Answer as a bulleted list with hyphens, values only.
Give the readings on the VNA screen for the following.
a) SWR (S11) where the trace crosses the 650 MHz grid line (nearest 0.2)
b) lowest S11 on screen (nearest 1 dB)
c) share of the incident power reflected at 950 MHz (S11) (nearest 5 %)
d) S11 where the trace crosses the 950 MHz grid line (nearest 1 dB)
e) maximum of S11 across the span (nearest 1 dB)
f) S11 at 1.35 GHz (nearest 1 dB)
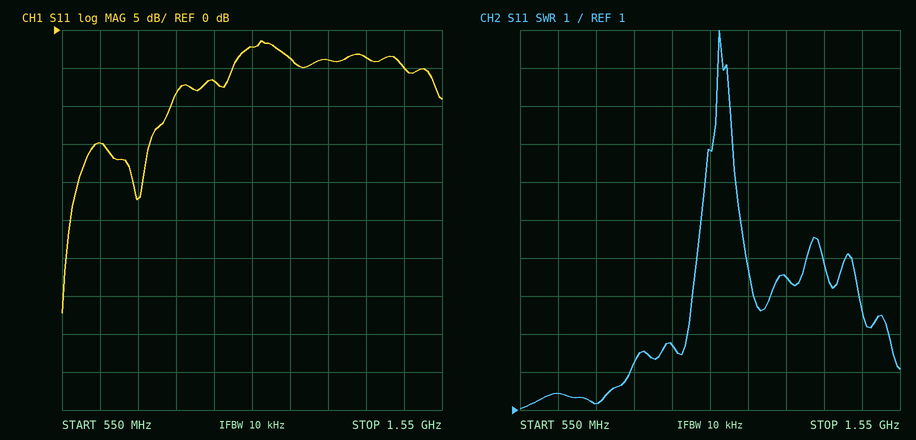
- 1.4
- -37 dB
- 20 %
- -7 dB
- -1 dB
- -4 dB
